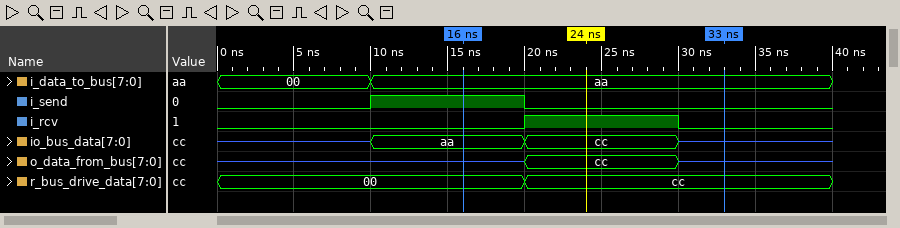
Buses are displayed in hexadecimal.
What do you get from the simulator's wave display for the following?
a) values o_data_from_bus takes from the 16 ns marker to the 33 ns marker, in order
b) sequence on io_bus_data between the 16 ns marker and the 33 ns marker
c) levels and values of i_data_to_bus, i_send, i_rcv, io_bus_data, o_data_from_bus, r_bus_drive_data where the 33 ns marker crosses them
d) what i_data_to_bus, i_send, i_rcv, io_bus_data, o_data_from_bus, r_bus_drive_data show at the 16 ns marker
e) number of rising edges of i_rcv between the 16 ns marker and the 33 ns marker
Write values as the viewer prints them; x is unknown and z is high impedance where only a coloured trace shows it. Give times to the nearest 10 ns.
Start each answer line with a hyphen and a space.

- z, cc, z
- aa, cc, z
- i_data_to_bus=aa, i_send=0, i_rcv=0, io_bus_data=z, o_data_from_bus=z, r_bus_drive_data=cc
- i_data_to_bus=aa, i_send=1, i_rcv=0, io_bus_data=aa, o_data_from_bus=z, r_bus_drive_data=00
- 1
